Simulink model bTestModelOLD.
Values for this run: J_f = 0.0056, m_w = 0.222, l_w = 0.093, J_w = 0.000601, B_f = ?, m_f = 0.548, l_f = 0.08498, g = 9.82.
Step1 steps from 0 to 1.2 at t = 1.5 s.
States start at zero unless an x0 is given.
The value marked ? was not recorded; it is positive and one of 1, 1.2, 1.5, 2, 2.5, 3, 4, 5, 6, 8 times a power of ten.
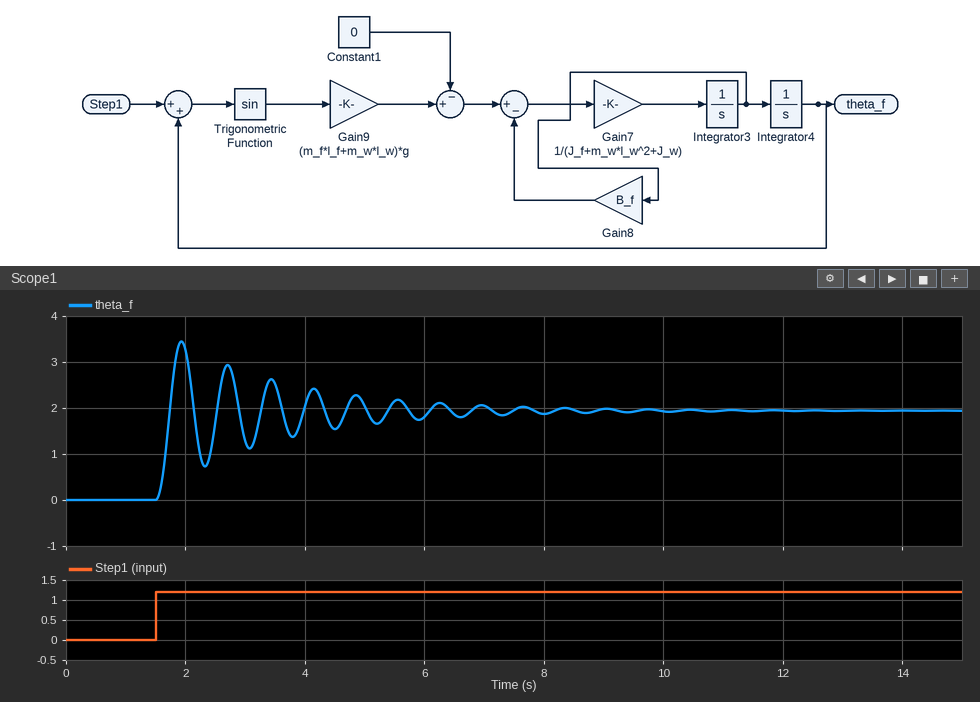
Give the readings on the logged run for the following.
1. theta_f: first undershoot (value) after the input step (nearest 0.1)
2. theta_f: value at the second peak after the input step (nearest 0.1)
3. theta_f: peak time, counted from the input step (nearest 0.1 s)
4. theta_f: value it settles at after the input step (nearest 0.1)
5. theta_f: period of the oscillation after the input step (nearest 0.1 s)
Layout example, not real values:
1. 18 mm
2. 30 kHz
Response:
1. 0.7
2. 2.9
3. 0.4 s
4. 1.9
5. 0.8 s
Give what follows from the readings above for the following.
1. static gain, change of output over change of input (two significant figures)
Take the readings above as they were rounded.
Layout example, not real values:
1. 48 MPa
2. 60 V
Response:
1. 1.6
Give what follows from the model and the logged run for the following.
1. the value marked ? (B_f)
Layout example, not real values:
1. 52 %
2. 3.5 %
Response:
1. 0.008
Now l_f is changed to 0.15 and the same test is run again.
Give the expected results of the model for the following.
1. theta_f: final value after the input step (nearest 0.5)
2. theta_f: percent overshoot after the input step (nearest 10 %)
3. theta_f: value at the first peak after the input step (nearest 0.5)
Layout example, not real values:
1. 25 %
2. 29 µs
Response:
1. 2.0
2. 80 %
3. 3.5
